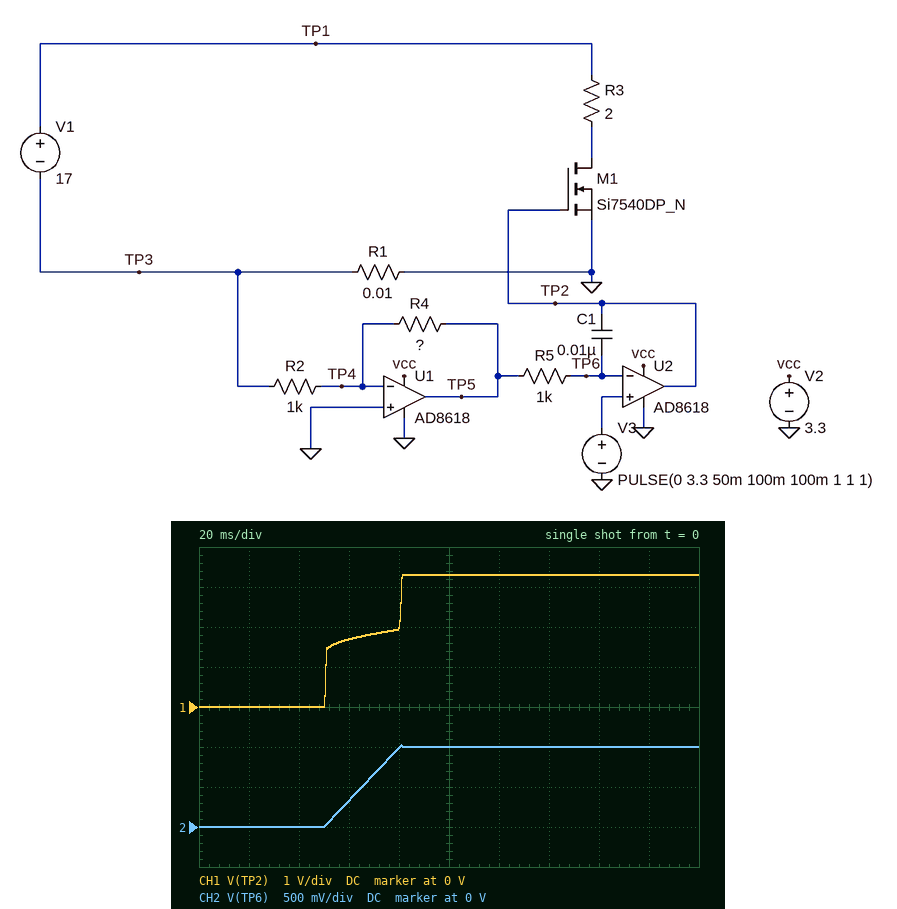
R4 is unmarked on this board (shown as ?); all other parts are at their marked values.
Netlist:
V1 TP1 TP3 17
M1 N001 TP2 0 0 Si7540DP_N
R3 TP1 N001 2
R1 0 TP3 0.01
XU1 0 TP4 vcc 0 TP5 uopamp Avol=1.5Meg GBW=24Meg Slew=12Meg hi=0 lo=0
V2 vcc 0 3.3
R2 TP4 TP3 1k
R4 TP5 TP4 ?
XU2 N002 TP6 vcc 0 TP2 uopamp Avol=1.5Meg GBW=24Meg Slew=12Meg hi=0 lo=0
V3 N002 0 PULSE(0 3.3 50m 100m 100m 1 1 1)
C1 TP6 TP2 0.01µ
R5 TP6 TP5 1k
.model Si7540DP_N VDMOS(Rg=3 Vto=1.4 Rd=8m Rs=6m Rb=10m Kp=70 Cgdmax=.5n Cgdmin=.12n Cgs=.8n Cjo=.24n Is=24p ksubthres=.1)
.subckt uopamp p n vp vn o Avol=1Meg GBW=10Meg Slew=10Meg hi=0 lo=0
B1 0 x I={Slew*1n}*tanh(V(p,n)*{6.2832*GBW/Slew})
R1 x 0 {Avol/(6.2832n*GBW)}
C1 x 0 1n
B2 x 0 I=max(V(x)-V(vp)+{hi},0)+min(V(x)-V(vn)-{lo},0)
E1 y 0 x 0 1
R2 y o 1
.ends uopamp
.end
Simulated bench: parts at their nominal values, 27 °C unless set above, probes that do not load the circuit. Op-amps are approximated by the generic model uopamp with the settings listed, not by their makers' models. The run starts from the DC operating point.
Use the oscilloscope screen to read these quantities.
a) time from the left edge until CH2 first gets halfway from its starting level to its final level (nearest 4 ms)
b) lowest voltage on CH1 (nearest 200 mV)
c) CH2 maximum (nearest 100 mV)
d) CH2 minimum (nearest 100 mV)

64 ms
0 V
1.0 V
0 V
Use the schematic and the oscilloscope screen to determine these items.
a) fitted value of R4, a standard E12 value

12 kΩ
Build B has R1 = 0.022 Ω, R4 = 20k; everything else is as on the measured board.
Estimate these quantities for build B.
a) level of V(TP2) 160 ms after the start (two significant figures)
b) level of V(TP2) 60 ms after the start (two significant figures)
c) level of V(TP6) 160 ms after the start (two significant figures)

1.9 V
1.5 V
3.3 V
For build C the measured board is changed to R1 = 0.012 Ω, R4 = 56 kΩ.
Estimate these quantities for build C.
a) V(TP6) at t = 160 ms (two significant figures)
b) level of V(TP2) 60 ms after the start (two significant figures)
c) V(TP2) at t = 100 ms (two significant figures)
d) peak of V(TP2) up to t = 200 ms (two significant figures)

3.3 V
1.5 V
1.7 V
1.8 V
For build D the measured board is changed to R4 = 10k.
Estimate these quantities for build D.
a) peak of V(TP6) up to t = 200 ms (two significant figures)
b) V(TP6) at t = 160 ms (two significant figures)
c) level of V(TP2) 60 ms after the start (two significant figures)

860 mV
840 mV
1.7 V
